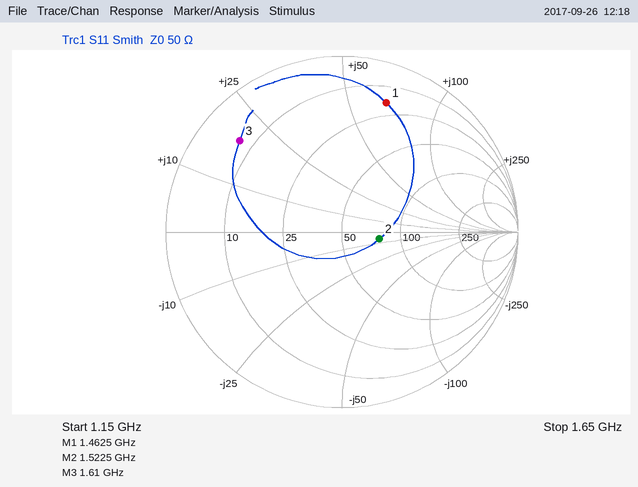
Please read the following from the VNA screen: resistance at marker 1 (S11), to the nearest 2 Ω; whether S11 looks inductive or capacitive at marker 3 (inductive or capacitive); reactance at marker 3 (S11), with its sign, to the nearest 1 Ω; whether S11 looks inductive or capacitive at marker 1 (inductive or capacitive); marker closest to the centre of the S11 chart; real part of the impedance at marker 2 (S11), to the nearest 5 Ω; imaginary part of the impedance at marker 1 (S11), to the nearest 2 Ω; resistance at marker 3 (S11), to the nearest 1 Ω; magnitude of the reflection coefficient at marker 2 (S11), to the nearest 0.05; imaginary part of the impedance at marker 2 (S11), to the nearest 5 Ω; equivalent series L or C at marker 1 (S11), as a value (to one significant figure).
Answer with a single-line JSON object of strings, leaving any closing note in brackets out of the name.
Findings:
{"resistance at marker 1 (S11), to the nearest 2 Ω": "18 Ω", "whether S11 looks inductive or capacitive at marker 3": "inductive", "reactance at marker 3 (S11), with its sign, to the nearest 1 Ω": "+19 Ω", "whether S11 looks inductive or capacitive at marker 1": "inductive", "marker closest to the centre of the S11 chart": "marker 2", "real part of the impedance at marker 2 (S11), to the nearest 5 Ω": "75 Ω", "imaginary part of the impedance at marker 1 (S11), to the nearest 2 Ω": "+66 Ω", "resistance at marker 3 (S11), to the nearest 1 Ω": "7 Ω", "magnitude of the reflection coefficient at marker 2 (S11), to the nearest 0.05": "0.20", "imaginary part of the impedance at marker 2 (S11), to the nearest 5 Ω": "-5 Ω", "equivalent series L or C at marker 1 (S11), as a value": "7 nH"}
